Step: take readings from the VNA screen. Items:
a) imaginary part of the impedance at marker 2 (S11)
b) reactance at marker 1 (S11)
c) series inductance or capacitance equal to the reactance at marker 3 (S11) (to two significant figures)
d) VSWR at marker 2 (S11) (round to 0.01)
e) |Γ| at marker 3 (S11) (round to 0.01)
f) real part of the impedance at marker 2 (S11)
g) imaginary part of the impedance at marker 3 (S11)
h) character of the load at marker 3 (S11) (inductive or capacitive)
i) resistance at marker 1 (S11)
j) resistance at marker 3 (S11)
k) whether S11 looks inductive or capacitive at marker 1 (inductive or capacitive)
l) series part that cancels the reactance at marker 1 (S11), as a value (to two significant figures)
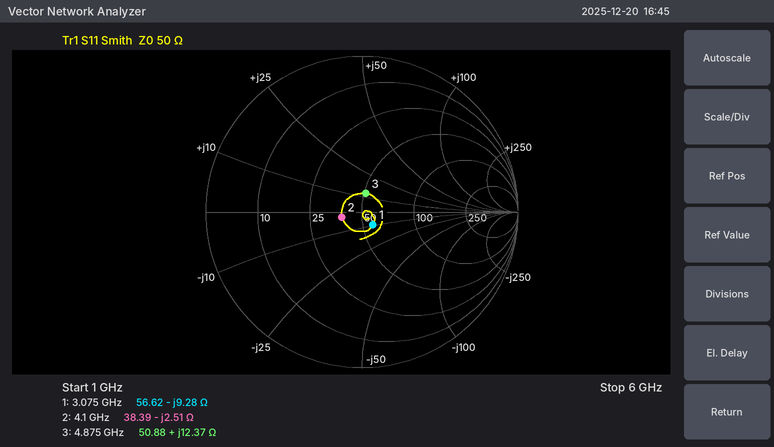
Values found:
-2.51 Ω
-9.28 Ω
400 pH
1.31
0.12
38.39 Ω
+12.37 Ω
inductive
56.62 Ω
50.88 Ω
capacitive
480 pH
